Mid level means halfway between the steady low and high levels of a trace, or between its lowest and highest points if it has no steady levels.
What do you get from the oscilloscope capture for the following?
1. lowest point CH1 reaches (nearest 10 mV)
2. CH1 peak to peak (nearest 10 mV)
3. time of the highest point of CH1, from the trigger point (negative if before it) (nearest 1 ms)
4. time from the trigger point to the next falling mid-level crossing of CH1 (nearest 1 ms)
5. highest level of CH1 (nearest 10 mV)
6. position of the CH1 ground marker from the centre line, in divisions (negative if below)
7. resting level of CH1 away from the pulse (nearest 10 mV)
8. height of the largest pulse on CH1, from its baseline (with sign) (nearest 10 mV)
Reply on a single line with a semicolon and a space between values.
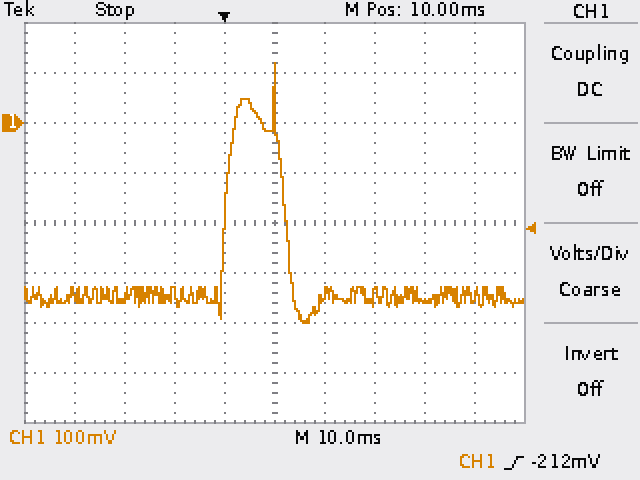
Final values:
-400 mV; 520 mV; +10 ms; 12 ms; 120 mV; +2.0 div; -350 mV; +470 mV
